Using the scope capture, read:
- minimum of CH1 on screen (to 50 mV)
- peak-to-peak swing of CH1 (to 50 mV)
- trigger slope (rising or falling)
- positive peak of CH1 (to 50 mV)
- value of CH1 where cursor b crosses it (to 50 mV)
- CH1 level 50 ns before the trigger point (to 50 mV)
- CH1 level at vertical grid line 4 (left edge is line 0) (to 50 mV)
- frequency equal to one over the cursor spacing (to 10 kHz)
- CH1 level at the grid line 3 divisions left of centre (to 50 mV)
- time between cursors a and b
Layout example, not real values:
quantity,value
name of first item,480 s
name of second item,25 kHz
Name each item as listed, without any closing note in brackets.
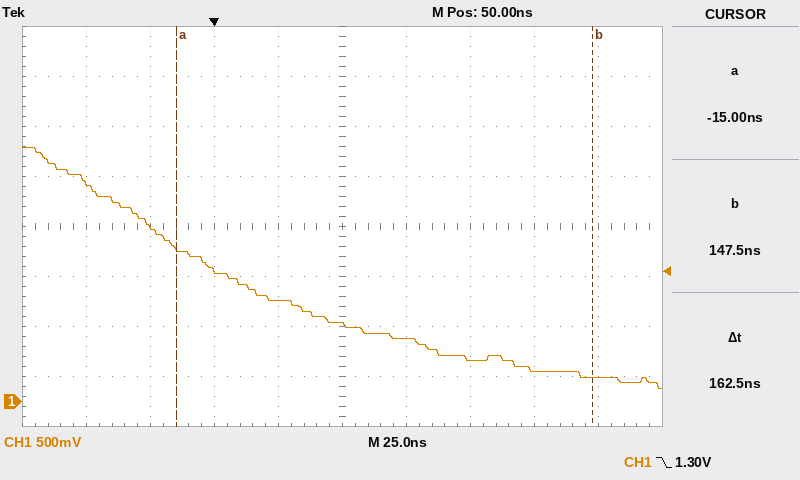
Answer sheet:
quantity,value
minimum of CH1 on screen,150 mV
peak-to-peak swing of CH1,2.40 V
trigger slope,falling
positive peak of CH1,2.55 V
value of CH1 where cursor b crosses it,250 mV
CH1 level 50 ns before the trigger point,2.20 V
CH1 level at vertical grid line 4 (left edge is line 0),1.00 V
frequency equal to one over the cursor spacing,6.15 MHz
CH1 level at the grid line 3 divisions left of centre,1.75 V
time between cursors a and b,162.5 ns
